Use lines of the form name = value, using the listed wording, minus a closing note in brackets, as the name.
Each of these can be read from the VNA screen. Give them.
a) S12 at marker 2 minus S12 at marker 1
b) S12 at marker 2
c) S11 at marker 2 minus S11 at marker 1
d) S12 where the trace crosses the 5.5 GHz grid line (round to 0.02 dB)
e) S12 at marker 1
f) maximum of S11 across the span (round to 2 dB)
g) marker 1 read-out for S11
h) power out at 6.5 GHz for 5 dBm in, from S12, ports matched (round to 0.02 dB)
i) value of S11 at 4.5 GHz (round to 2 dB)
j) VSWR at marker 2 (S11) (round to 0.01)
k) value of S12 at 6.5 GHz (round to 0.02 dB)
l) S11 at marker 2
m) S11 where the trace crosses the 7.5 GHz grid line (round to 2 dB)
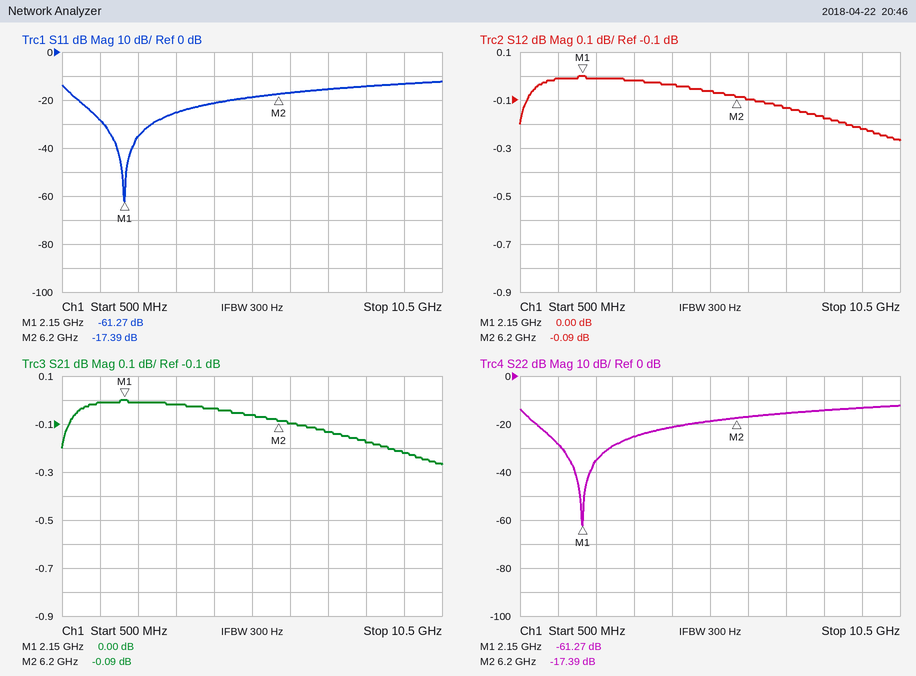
S12 at marker 2 minus S12 at marker 1 = -0.09 dB
S12 at marker 2 = -0.09 dB
S11 at marker 2 minus S11 at marker 1 = 43.88 dB
S12 where the trace crosses the 5.5 GHz grid line = -0.06 dB
S12 at marker 1 = 0.00 dB
maximum of S11 across the span = -12 dB
marker 1 read-out for S11 = -61.27 dB
power out at 6.5 GHz for 5 dBm in, from S12, ports matched = 4.90 dBm
value of S11 at 4.5 GHz = -22 dB
VSWR at marker 2 (S11) = 1.31
value of S12 at 6.5 GHz = -0.10 dB
S11 at marker 2 = -17.39 dB
S11 where the trace crosses the 7.5 GHz grid line = -16 dB
